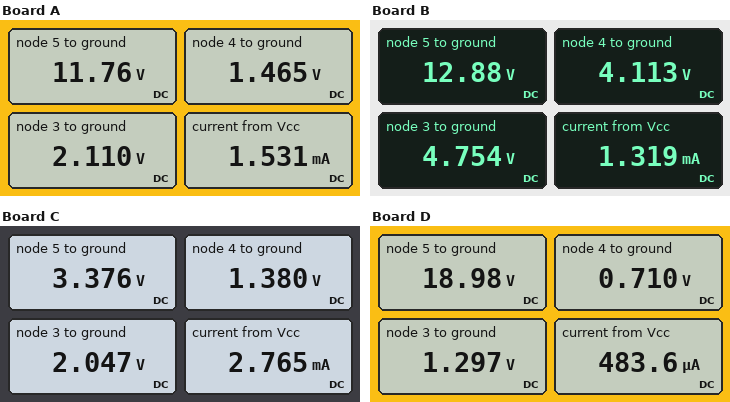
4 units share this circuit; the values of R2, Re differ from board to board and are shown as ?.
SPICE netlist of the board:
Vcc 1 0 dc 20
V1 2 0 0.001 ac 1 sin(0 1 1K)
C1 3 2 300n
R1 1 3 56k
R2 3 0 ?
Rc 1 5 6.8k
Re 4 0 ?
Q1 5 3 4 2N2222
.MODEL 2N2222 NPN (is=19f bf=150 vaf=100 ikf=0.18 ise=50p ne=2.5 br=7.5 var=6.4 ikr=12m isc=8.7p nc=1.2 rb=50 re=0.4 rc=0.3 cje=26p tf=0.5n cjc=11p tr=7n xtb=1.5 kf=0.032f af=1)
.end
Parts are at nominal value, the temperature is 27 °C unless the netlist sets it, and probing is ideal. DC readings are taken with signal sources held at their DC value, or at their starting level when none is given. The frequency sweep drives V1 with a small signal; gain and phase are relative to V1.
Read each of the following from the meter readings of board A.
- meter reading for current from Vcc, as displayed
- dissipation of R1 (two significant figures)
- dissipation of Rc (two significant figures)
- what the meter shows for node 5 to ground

1.531 mA
5.7 mW
10 mW
11.76 V
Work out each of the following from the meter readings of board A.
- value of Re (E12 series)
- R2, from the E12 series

1.2 kΩ
6.8 kΩ
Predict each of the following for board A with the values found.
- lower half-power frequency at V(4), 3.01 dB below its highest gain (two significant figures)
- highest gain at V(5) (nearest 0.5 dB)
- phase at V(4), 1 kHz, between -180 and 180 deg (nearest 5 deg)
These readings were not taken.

91 Hz
15.0 dB
5 deg
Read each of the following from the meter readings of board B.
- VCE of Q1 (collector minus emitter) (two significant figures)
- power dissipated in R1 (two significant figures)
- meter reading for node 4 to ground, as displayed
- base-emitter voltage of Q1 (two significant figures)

8.8 V
4.2 mW
4.113 V
640 mV
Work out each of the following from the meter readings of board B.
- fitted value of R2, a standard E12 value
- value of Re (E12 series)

18 kΩ
3.9 kΩ
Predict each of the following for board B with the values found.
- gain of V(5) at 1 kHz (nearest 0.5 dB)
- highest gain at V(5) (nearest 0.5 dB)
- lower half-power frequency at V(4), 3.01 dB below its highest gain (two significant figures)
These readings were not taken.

4.5 dB
4.5 dB
40 Hz
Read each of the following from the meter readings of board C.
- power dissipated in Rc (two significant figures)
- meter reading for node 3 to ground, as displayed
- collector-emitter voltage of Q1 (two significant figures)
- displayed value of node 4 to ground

41 mW
2.047 V
2.0 V
1.380 V
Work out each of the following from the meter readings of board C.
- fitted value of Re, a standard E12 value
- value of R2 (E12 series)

560 Ω
6.8 kΩ
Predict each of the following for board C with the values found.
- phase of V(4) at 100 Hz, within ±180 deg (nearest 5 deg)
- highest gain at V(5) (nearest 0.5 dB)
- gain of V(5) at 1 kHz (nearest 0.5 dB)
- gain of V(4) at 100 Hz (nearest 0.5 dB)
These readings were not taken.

45 deg
21.5 dB
21.5 dB
-3.0 dB
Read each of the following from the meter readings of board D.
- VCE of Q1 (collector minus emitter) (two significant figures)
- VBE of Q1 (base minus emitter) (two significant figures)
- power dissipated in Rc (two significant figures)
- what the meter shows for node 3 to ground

18 V
590 mV
150 µW
1.297 V
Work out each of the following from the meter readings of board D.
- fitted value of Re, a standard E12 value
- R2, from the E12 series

4.7 kΩ
3.9 kΩ
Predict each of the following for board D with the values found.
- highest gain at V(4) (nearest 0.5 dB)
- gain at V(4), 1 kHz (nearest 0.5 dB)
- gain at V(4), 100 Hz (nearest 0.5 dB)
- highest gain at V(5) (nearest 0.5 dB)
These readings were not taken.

-0.5 dB
-0.5 dB
-5.5 dB
3.0 dB
